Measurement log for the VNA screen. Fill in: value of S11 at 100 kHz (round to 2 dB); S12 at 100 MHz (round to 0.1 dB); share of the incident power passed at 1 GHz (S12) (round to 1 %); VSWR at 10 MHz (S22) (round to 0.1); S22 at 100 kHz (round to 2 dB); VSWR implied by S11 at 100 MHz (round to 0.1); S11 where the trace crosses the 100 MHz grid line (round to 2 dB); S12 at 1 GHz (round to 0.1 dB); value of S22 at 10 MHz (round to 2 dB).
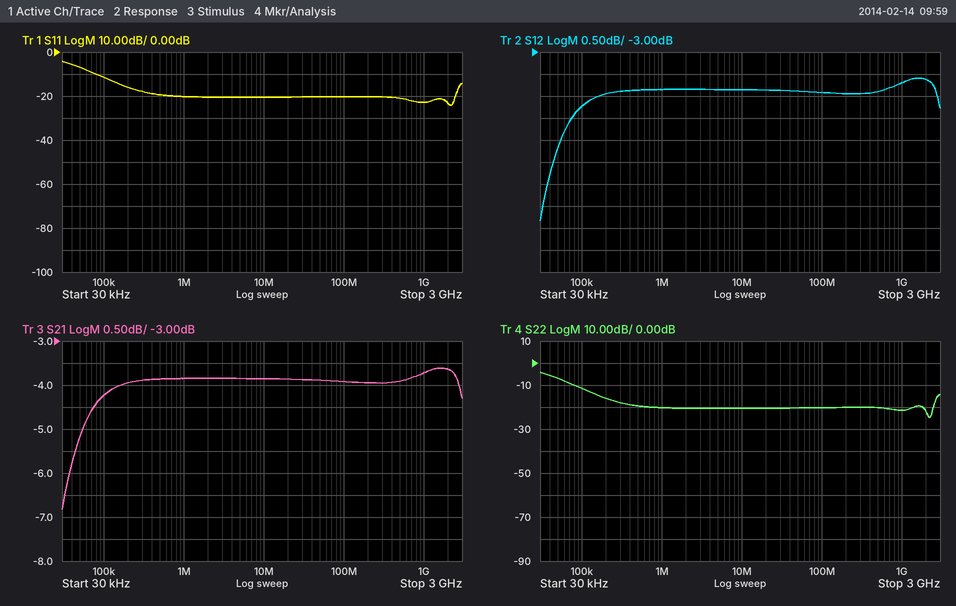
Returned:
-12 dB
-3.9 dB
43 %
1.2
-12 dB
1.2
-20 dB
-3.7 dB
-20 dB
